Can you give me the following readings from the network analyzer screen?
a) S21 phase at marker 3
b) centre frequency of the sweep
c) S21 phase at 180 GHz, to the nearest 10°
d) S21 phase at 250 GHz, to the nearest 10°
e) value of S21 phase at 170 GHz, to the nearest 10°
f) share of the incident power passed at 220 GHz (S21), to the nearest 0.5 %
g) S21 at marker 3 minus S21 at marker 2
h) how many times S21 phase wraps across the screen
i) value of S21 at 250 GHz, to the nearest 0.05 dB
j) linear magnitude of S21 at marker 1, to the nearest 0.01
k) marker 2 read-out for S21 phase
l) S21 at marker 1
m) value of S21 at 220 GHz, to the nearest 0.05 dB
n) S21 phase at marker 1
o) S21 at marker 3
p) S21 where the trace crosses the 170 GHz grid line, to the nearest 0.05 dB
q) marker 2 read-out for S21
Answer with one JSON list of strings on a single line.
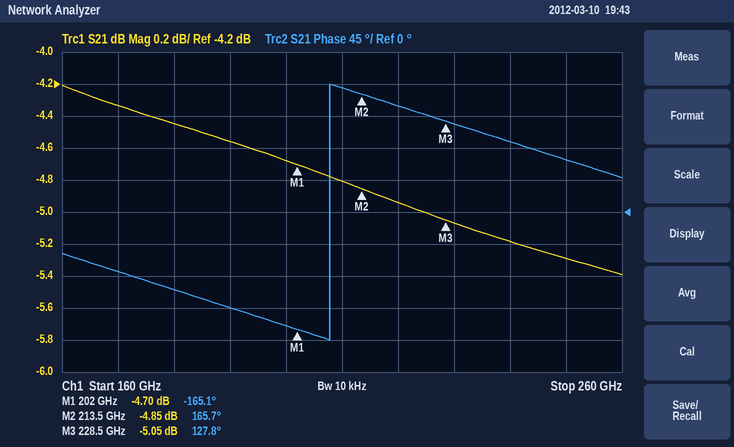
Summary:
["127.8°", "210 GHz", "-110°", "70°", "-80°", "32.0 %", "-0.20 dB", "1", "-5.30 dB", "0.58", "165.7°", "-4.70 dB", "-4.95 dB", "-165.1°", "-5.05 dB", "-4.35 dB", "-4.85 dB"]
